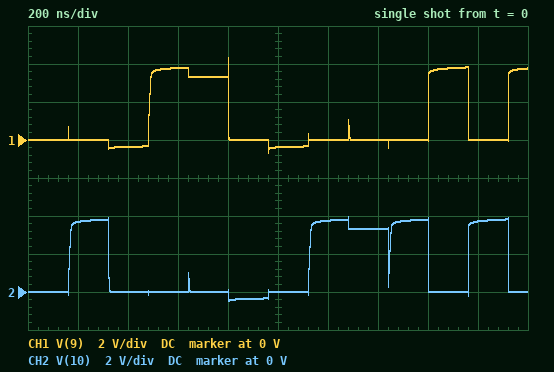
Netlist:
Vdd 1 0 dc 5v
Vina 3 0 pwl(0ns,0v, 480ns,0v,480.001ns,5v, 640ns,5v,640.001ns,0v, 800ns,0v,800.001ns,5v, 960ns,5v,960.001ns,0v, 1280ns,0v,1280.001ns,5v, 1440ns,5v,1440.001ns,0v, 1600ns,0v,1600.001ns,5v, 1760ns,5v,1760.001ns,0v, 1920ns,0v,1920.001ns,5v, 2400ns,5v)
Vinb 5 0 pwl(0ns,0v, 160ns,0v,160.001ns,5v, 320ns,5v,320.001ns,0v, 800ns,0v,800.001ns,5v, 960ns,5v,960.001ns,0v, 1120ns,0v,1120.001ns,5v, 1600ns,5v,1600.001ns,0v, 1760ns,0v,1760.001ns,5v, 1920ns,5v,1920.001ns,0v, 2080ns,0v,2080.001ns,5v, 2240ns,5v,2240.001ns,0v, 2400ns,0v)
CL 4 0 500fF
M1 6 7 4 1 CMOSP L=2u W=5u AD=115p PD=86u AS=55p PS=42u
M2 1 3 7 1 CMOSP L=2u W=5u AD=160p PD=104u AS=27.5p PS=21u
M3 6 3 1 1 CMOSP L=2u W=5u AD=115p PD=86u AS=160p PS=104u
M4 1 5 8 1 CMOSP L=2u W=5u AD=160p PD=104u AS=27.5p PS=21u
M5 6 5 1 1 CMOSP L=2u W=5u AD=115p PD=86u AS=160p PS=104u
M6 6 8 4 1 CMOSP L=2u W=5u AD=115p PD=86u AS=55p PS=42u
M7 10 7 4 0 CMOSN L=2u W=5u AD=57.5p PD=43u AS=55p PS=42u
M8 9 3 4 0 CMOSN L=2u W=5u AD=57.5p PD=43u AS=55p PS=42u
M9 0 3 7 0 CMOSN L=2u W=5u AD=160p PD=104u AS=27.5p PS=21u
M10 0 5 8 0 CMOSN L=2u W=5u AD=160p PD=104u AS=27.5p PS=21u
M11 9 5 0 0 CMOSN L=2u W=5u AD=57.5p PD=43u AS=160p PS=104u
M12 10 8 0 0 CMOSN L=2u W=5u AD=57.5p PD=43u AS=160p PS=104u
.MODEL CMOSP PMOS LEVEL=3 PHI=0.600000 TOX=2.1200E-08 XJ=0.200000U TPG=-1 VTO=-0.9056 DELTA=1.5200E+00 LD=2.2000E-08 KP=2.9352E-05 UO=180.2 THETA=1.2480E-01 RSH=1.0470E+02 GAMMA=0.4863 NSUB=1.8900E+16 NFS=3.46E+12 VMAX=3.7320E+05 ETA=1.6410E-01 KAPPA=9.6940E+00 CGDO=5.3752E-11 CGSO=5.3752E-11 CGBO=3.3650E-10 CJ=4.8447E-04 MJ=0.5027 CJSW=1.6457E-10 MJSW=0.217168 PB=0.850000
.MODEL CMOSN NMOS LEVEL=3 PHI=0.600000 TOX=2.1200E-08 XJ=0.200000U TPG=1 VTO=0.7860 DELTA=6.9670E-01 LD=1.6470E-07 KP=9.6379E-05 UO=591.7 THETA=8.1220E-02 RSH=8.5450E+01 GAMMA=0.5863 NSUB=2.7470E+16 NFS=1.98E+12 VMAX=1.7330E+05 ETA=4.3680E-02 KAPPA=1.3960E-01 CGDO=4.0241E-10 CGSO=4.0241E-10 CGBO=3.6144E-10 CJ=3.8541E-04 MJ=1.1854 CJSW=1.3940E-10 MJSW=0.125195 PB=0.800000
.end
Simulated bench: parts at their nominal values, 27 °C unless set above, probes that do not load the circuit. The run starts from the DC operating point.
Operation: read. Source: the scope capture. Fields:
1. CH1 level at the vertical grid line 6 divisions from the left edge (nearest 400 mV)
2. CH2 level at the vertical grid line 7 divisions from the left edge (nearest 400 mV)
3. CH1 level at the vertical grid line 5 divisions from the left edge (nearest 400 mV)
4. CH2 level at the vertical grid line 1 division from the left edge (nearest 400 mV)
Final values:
0 V
3.2 V
-400 mV
3.6 V
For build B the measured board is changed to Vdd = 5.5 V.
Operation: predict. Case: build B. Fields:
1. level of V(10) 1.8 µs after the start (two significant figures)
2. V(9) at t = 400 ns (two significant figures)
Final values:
4.2 V
-360 mV
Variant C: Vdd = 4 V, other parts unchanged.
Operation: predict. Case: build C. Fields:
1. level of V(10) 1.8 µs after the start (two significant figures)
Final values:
2.8 V
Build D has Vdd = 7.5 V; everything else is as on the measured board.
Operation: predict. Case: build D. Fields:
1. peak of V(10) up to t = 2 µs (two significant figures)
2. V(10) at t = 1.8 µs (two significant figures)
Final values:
6.2 V
6.0 V
